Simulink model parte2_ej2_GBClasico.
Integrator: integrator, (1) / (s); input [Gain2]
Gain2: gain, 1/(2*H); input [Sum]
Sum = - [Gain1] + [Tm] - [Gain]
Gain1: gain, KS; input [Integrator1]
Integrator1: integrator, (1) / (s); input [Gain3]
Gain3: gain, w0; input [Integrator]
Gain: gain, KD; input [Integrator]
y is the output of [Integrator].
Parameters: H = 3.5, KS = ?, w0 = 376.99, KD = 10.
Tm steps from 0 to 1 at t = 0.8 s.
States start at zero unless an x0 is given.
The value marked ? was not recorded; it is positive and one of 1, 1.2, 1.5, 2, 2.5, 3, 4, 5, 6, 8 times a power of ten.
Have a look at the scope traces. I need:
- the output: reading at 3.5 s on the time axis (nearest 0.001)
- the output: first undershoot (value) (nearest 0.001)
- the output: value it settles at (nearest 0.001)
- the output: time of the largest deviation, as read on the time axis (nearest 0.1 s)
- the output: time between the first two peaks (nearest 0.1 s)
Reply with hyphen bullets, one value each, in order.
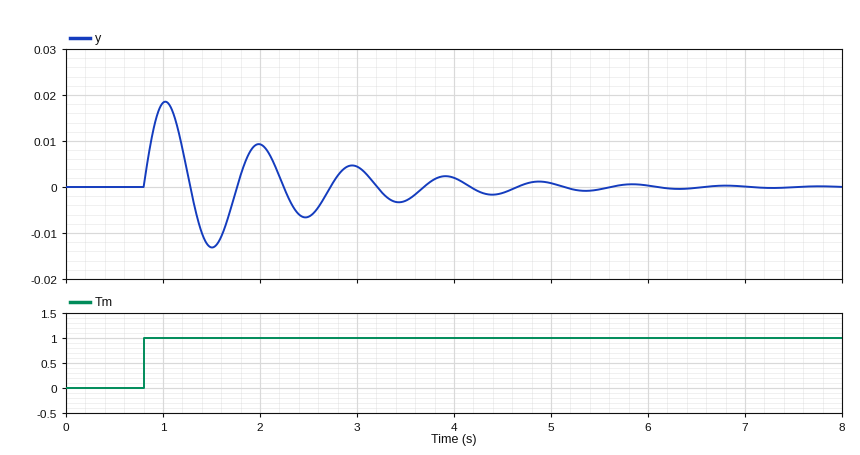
- -0.003
- -0.013
- 0.000
- 1.0 s
- 1.0 s
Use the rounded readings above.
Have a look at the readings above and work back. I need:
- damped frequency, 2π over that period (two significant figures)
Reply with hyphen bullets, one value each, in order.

- 6.3 rad/s
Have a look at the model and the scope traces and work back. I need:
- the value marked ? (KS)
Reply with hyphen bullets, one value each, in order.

- 0.8
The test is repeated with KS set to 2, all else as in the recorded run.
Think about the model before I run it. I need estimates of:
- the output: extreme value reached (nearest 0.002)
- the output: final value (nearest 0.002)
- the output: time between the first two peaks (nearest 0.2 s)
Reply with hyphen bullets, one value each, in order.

- 0.012
- 0.000
- 0.6 s
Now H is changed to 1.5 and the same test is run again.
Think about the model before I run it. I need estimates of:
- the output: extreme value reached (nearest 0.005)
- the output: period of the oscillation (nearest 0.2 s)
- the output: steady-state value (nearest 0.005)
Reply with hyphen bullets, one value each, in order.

- 0.025
- 0.6 s
- 0.000
